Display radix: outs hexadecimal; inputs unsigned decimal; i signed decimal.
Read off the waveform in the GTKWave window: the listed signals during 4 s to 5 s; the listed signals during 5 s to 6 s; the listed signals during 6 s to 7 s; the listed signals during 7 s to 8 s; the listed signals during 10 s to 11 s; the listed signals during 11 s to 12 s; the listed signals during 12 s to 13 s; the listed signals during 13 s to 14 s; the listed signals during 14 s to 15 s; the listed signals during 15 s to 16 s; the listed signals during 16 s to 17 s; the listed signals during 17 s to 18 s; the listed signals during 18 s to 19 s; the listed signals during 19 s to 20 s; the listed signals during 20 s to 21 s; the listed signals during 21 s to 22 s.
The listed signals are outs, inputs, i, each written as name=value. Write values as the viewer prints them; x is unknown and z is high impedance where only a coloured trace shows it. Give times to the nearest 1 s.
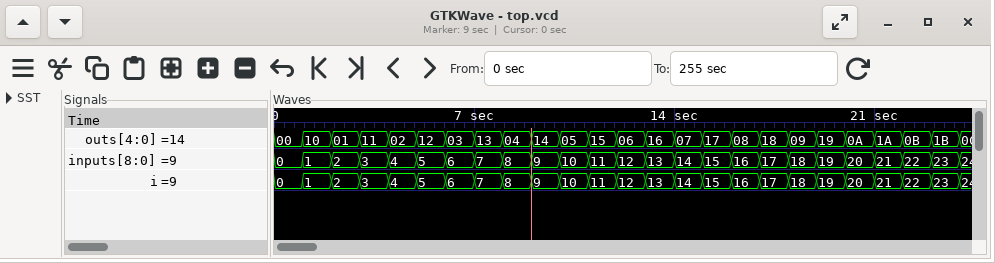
outs=02, inputs=4, i=4
outs=12, inputs=5, i=5
outs=03, inputs=6, i=6
outs=13, inputs=7, i=7
outs=05, inputs=10, i=10
outs=15, inputs=11, i=11
outs=06, inputs=12, i=12
outs=16, inputs=13, i=13
outs=07, inputs=14, i=14
outs=17, inputs=15, i=15
outs=08, inputs=16, i=16
outs=18, inputs=17, i=17
outs=09, inputs=18, i=18
outs=19, inputs=19, i=19
outs=0A, inputs=20, i=20
outs=1A, inputs=21, i=21
